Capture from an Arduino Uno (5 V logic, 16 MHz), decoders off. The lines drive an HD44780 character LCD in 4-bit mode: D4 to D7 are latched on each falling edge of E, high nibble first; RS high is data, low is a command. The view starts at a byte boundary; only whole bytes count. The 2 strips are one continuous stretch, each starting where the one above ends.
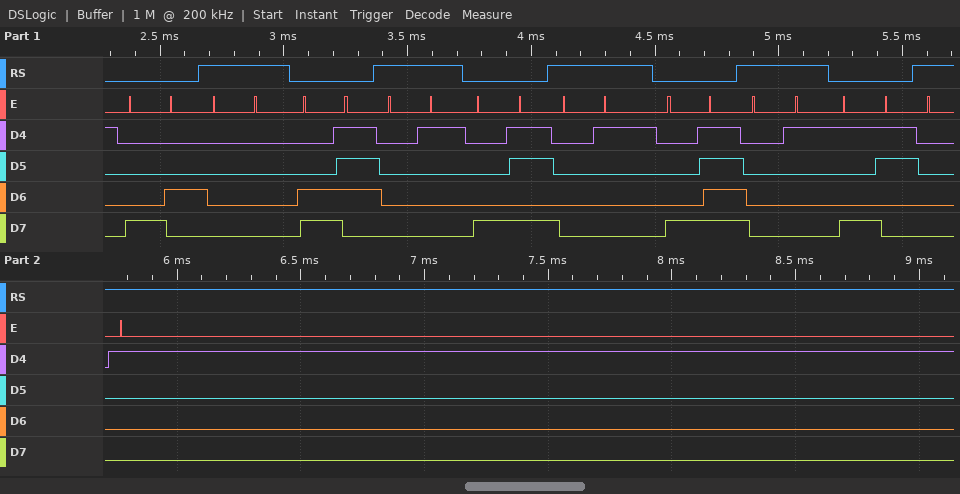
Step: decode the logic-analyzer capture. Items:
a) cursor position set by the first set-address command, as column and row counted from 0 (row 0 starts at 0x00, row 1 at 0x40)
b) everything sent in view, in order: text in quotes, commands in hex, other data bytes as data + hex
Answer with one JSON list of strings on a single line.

["column 4, row 0", "0x84 data 00 0xC7 data 01 0x8B data 01 0x8F data 01 0x93 data 01"]
